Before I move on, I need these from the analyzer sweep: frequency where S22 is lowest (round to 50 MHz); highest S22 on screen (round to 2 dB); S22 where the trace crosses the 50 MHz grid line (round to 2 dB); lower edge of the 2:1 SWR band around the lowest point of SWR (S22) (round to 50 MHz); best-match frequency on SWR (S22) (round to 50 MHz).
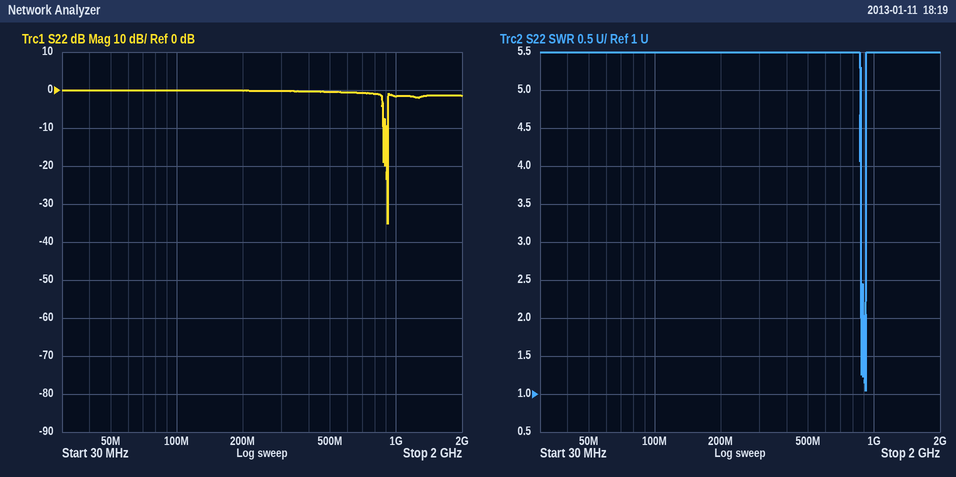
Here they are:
900 MHz
0 dB
0 dB
900 MHz
900 MHz
